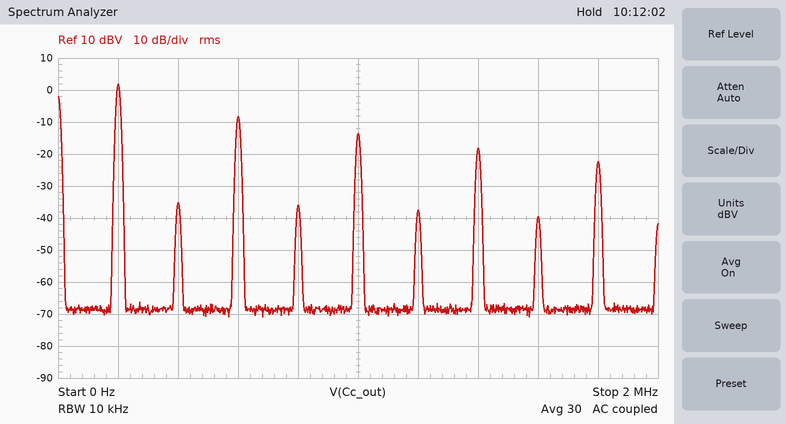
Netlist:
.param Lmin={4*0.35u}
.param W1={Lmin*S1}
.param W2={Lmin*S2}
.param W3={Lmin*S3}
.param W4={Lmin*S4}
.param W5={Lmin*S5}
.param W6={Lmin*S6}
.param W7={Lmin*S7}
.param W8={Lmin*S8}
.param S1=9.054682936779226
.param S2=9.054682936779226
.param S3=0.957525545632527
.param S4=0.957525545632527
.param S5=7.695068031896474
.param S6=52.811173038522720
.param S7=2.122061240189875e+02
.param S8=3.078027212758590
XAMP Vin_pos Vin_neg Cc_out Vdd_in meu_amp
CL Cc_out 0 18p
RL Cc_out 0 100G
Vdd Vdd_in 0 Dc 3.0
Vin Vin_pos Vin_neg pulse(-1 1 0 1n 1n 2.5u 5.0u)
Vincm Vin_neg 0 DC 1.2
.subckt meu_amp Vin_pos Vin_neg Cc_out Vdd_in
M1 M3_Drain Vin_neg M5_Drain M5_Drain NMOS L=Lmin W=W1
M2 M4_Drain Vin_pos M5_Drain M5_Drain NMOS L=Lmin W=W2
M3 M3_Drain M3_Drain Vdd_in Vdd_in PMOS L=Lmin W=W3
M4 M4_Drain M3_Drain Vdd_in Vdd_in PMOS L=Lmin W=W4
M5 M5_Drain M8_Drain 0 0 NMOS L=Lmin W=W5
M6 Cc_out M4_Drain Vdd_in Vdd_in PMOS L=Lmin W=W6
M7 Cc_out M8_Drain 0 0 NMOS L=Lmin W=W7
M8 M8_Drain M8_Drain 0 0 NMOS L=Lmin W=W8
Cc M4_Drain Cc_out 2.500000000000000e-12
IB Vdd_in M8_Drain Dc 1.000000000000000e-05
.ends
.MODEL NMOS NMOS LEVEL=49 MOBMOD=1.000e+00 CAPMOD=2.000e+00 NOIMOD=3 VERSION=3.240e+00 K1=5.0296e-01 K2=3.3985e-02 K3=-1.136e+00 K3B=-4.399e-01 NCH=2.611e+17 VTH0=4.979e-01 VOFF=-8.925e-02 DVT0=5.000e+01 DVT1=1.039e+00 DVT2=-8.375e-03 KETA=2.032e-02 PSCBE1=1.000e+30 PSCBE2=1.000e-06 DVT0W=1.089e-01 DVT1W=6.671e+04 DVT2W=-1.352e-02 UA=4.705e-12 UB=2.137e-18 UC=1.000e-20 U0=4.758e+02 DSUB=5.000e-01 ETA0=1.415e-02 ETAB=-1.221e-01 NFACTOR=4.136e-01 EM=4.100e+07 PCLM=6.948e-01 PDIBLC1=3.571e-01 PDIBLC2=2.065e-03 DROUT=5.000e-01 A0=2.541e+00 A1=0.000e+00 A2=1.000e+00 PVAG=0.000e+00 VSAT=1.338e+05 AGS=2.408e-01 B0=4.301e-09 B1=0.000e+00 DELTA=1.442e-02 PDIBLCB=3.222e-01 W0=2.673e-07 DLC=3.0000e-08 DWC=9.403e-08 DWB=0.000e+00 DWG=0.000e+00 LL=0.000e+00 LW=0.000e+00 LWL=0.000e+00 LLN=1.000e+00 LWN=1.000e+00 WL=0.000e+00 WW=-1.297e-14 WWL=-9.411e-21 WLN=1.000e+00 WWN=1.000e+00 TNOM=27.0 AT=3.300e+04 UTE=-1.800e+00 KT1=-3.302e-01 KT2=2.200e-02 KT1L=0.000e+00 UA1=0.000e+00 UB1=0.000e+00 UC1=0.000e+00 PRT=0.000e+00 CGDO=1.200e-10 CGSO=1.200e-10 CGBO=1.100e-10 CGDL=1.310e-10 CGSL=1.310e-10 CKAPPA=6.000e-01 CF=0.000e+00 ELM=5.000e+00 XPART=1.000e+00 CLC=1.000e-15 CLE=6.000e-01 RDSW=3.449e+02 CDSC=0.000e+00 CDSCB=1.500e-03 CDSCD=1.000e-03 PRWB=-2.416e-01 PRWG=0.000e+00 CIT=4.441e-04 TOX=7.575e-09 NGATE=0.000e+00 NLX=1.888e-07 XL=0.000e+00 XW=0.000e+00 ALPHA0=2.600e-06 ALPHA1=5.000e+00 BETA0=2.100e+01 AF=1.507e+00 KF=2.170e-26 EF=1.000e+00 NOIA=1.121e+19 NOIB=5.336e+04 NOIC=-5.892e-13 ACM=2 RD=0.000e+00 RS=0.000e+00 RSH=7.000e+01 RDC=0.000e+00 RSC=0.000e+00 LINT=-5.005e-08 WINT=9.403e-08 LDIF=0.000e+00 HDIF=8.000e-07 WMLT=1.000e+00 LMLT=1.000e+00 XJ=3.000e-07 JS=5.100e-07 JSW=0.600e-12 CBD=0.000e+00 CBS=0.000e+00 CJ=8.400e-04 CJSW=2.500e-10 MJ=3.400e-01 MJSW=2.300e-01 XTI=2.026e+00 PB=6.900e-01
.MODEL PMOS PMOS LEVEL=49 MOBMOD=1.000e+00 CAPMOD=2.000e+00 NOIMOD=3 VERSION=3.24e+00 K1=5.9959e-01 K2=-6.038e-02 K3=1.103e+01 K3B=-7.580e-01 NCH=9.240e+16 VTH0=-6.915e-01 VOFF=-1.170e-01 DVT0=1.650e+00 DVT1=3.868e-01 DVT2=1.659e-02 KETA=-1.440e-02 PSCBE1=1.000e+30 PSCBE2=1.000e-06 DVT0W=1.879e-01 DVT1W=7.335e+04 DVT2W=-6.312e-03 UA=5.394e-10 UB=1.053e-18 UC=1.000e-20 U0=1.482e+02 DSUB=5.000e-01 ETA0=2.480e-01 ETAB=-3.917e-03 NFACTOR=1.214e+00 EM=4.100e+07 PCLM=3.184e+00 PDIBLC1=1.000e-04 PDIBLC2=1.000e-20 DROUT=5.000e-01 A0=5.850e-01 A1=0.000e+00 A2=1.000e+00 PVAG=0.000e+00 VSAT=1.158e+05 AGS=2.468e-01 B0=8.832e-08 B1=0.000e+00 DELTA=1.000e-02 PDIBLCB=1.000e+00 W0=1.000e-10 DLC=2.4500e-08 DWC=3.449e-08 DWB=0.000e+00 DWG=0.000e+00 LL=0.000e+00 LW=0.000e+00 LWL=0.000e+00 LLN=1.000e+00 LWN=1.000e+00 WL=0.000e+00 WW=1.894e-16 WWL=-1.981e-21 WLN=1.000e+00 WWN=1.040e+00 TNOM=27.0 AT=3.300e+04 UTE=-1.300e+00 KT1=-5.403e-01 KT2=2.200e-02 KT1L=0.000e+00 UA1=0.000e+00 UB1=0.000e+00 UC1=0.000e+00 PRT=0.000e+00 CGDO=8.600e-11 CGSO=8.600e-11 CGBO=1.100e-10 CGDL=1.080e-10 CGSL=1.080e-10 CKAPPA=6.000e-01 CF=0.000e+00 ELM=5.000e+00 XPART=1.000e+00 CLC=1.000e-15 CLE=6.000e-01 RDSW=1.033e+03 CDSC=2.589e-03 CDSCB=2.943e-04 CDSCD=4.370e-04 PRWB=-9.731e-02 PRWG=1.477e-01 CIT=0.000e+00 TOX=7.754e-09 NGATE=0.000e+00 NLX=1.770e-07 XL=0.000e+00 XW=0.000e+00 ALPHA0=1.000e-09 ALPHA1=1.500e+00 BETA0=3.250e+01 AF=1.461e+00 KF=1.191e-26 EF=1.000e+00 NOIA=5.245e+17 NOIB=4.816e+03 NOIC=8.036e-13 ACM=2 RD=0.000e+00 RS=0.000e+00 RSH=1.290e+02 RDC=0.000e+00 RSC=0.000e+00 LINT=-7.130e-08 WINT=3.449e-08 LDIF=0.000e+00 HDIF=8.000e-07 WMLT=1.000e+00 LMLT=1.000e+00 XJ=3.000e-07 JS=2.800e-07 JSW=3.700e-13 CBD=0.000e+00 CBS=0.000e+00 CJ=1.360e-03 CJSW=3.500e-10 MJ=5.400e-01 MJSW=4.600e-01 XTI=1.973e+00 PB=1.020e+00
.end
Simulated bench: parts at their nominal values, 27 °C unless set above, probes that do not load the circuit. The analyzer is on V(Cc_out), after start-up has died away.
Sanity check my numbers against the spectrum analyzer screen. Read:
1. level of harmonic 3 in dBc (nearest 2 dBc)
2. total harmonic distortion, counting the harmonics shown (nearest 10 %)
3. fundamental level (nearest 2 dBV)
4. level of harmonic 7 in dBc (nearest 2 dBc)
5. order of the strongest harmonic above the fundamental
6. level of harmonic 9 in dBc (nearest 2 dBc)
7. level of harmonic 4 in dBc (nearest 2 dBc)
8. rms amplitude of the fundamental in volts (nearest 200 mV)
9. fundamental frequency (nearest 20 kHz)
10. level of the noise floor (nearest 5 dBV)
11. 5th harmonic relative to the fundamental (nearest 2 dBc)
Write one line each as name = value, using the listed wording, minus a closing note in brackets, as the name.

level of harmonic 3 in dBc = -10 dBc
total harmonic distortion, counting the harmonics shown = 40 %
fundamental level = 2 dBV
level of harmonic 7 in dBc = -20 dBc
order of the strongest harmonic above the fundamental = 3
level of harmonic 9 in dBc = -24 dBc
level of harmonic 4 in dBc = -38 dBc
rms amplitude of the fundamental in volts = 1.2 V
fundamental frequency = 200 kHz
level of the noise floor = -70 dBV
5th harmonic relative to the fundamental = -16 dBc
